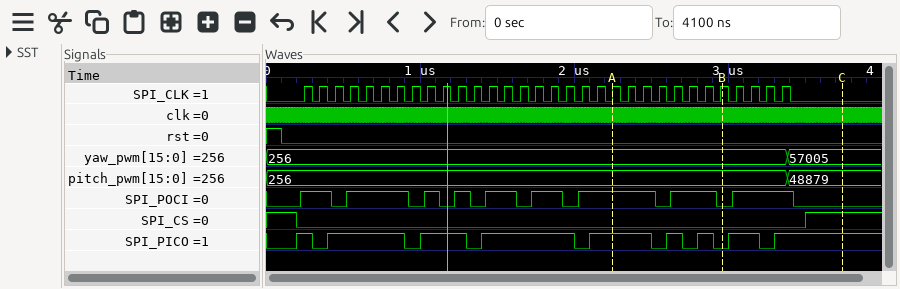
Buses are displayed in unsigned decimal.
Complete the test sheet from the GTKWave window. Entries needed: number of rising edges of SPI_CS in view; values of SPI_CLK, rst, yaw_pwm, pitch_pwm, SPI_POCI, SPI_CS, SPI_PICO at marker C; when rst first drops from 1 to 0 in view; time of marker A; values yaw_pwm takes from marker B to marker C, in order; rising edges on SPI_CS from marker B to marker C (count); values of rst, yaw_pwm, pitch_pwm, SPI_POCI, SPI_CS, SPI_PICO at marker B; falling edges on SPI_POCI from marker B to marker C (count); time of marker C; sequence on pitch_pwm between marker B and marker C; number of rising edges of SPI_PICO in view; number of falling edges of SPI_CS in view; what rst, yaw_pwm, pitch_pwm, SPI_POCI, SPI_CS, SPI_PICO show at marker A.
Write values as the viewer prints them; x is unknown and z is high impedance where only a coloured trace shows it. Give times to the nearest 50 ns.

1
SPI_CLK=0, rst=0, yaw_pwm=57005, pitch_pwm=48879, SPI_POCI=0, SPI_CS=1, SPI_PICO=1
100 ns
2250 ns
256, 57005
1
rst=0, yaw_pwm=256, pitch_pwm=256, SPI_POCI=0, SPI_CS=0, SPI_PICO=0
1
3750 ns
256, 48879
9
1
rst=0, yaw_pwm=256, pitch_pwm=256, SPI_POCI=1, SPI_CS=0, SPI_PICO=1
